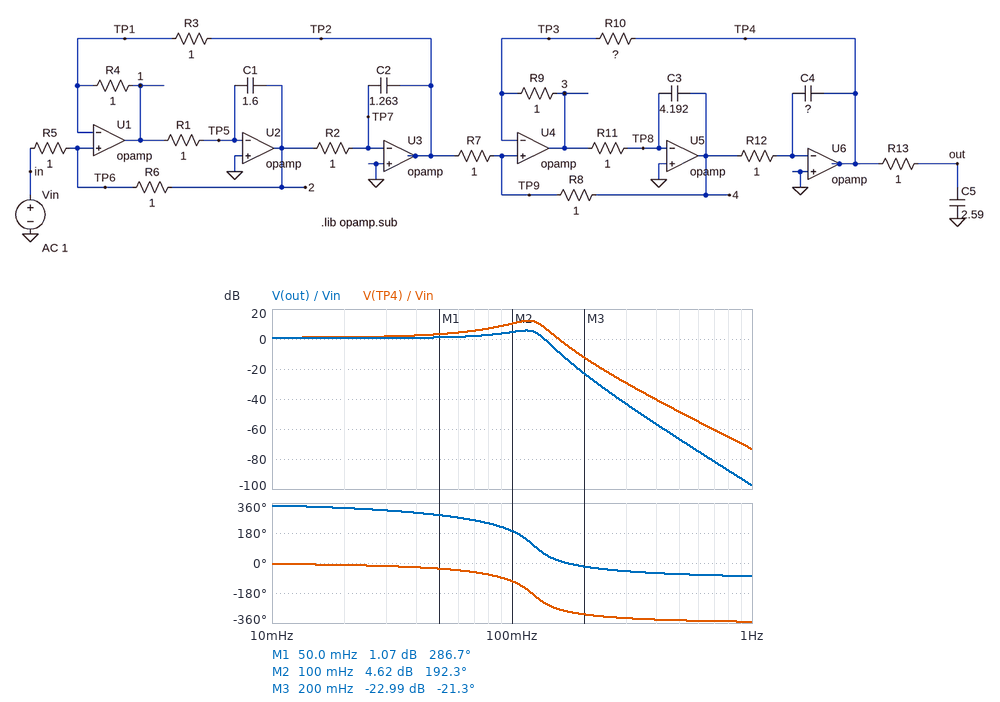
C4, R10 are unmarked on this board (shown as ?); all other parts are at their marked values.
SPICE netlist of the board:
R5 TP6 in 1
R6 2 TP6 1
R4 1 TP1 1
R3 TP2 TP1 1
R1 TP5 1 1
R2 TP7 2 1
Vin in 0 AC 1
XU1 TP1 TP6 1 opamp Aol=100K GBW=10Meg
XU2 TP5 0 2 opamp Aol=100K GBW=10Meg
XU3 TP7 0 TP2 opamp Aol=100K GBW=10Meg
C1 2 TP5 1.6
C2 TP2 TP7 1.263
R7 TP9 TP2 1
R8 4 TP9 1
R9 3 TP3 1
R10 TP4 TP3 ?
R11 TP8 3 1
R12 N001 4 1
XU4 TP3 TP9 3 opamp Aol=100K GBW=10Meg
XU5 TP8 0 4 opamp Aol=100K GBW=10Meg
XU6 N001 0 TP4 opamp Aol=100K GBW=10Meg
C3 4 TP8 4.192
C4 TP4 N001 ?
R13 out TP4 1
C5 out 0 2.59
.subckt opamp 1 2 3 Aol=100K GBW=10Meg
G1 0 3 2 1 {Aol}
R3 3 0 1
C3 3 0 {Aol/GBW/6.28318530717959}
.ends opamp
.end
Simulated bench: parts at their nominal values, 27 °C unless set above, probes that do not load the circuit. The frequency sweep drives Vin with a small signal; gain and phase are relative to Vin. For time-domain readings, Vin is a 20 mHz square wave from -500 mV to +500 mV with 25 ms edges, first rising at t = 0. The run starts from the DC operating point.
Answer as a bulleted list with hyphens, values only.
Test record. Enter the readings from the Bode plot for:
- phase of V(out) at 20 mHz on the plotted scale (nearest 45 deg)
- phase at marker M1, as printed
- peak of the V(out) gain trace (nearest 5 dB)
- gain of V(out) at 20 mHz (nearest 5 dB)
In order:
- 315 deg
- 286.7 deg
- 5 dB
- 0 dB
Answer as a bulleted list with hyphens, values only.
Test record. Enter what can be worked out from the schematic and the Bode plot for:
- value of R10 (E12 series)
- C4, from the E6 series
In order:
- 1.2 Ω
- 330 mF
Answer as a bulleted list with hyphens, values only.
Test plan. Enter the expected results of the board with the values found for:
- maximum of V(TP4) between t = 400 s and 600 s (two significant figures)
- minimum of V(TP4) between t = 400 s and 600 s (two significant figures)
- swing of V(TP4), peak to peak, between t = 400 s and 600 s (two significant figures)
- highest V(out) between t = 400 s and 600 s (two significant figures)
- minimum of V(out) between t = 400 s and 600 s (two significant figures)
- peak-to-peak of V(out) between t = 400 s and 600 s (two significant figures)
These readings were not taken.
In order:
- 1.3 V
- -1.3 V
- 2.6 V
- 840 mV
- -840 mV
- 1.7 V
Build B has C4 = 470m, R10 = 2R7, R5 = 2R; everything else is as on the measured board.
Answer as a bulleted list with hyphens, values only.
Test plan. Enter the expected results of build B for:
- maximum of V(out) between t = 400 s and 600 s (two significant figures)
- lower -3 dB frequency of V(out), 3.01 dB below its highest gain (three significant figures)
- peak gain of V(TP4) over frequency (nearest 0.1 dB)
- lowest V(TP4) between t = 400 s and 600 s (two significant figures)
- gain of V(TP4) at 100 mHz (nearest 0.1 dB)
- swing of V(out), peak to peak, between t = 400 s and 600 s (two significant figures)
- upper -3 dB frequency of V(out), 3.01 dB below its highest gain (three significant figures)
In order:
- 1.1 V
- 46.1 mHz
- 10.8 dB
- -1.4 V
- -0.6 dB
- 2.2 V
- 76.4 mHz
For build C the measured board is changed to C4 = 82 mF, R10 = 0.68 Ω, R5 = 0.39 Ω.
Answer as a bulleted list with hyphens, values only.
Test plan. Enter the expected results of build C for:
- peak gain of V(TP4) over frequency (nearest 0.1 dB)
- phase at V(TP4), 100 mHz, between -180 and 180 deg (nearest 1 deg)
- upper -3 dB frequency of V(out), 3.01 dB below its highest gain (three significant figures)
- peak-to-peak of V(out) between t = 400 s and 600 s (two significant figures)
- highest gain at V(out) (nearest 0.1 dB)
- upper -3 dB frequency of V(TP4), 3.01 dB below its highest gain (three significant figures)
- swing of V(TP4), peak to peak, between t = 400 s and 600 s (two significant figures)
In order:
- 8.9 dB
- -68 deg
- 126 mHz
- 1.5 V
- 3.1 dB
- 134 mHz
- 2.3 V
